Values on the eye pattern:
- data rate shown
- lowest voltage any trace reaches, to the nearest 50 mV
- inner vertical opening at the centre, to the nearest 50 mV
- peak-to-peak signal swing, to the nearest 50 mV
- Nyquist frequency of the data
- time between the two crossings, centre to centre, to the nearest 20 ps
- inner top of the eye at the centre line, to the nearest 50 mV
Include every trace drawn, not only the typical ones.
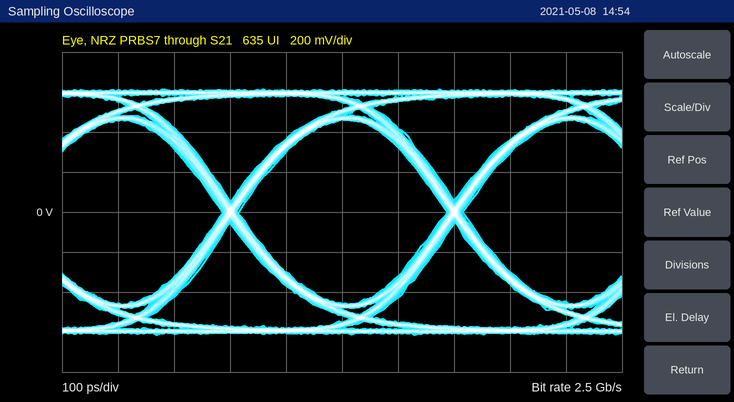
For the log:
2.5 Gb/s
-600 mV
900 mV
1.25 V
1.25 GHz
400 ps
450 mV
